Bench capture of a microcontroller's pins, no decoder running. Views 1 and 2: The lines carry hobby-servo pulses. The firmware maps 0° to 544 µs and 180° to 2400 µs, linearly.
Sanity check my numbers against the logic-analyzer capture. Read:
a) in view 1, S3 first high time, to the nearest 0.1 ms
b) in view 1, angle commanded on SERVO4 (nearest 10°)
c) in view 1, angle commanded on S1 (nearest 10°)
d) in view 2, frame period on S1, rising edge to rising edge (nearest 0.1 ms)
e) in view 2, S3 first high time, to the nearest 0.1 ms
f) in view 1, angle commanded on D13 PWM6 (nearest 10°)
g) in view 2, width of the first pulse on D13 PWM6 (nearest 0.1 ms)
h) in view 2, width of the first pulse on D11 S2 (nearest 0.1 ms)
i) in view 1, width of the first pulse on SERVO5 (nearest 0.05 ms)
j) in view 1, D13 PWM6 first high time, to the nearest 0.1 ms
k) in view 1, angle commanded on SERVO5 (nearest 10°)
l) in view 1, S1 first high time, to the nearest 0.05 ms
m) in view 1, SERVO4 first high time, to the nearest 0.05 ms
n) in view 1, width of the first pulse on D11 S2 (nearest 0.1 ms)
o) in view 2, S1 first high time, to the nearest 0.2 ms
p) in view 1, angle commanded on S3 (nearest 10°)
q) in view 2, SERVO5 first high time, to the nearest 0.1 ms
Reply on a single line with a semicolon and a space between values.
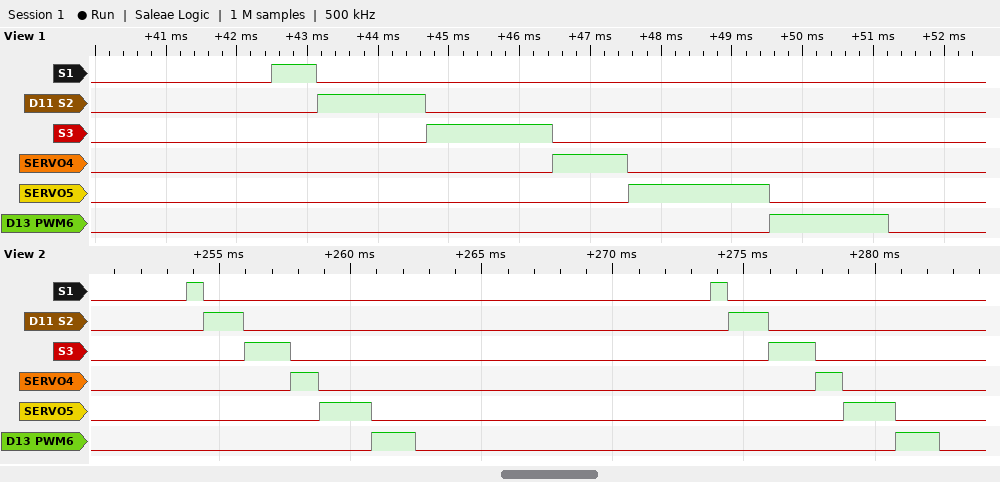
1.8 ms; 50°; 10°; 20.0 ms; 1.8 ms; 110°; 1.7 ms; 1.5 ms; 2.00 ms; 1.7 ms; 140°; 0.65 ms; 1.05 ms; 1.5 ms; 0.6 ms; 120°; 2.0 ms
